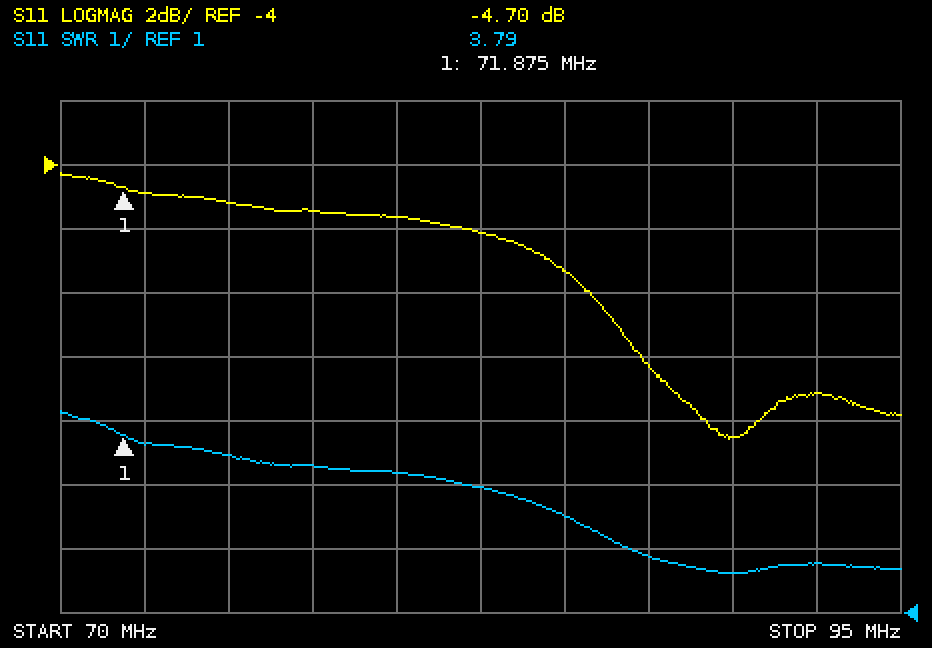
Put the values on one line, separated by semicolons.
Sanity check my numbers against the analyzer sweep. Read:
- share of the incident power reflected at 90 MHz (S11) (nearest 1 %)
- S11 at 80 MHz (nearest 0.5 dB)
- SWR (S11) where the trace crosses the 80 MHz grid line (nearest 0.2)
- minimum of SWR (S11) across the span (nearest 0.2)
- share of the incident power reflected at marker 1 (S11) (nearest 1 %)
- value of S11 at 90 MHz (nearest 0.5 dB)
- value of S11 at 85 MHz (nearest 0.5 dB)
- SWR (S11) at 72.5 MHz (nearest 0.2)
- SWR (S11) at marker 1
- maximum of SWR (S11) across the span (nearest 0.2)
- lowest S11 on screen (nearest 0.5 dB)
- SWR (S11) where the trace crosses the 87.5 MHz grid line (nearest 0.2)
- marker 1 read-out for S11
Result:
6 %; -5.5 dB; 3.2; 1.6; 34 %; -12.5 dB; -7.5 dB; 3.6; 3.79; 4.2; -12.5 dB; 1.8; -4.70 dB
